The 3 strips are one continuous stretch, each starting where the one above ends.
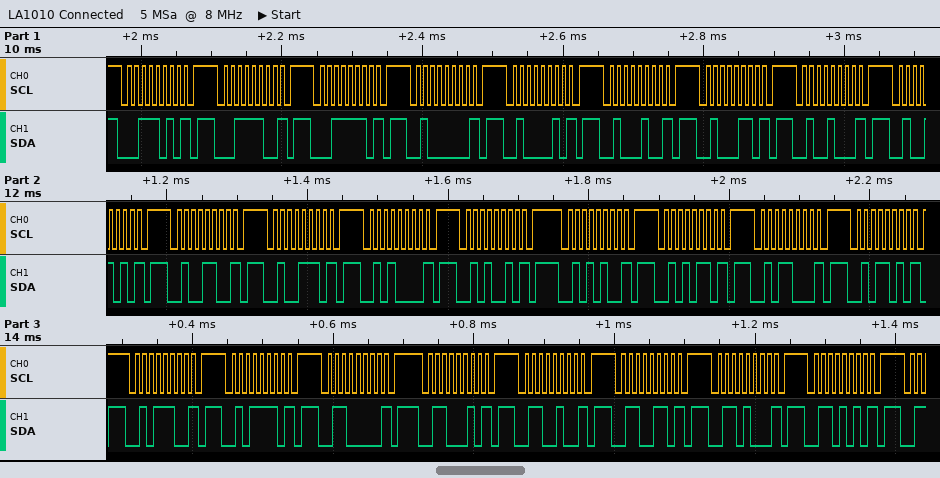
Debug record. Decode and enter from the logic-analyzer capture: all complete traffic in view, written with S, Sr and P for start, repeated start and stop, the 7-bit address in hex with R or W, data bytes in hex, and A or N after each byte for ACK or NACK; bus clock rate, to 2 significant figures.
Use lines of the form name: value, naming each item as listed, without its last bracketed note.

all complete traffic in view, written with S, Sr and P for start, repeated start and stop, the 7-bit address in hex with R or W, data bytes in hex, and A or N after each byte for ACK or NACK: S 1DW N P S 1EW N P S 1FW N P S 20W N P S 21W N P S 22W N P S 23W N P S 24W N P S 25W N P S 26W N P S 27W N P S 28W N P S 29W N P S 2AW N P S 2BW N P S 2CW N P S 2DW N P S 2EW N P S 2FW N P S 30W N P S 31W N P S 32W N P S 33W N P S 34W N P S 35W N P
bus clock rate, to 2 significant figures: 100 kHz
